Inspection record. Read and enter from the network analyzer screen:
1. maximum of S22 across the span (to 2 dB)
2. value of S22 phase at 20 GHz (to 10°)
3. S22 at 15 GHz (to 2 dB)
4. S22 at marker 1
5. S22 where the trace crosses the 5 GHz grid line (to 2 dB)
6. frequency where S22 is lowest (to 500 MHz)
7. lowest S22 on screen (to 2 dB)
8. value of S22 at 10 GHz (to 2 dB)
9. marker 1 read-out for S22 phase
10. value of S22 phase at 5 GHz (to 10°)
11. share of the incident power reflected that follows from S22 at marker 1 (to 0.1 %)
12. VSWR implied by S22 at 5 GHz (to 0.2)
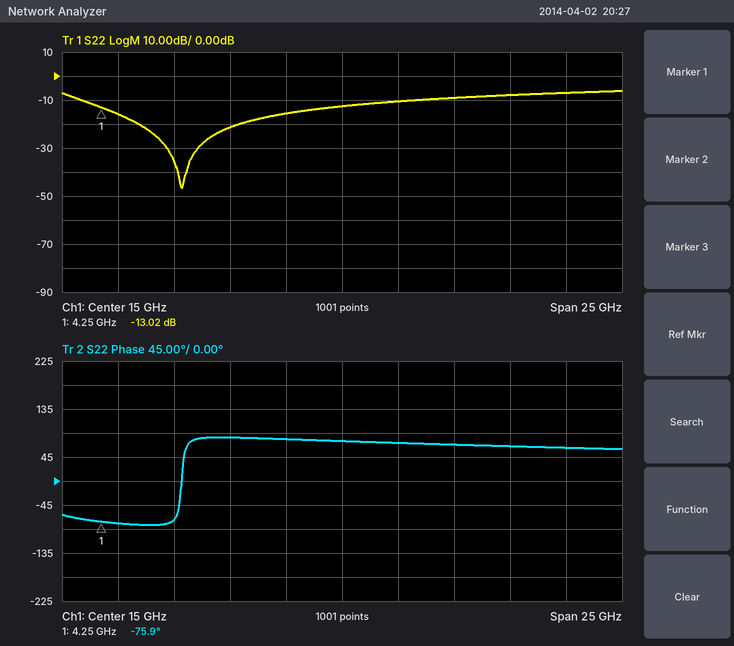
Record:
-6 dB
70°
-12 dB
-13.02 dB
-16 dB
8.0 GHz
-46 dB
-22 dB
-75.9°
-80°
5.0 %
1.4
